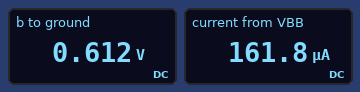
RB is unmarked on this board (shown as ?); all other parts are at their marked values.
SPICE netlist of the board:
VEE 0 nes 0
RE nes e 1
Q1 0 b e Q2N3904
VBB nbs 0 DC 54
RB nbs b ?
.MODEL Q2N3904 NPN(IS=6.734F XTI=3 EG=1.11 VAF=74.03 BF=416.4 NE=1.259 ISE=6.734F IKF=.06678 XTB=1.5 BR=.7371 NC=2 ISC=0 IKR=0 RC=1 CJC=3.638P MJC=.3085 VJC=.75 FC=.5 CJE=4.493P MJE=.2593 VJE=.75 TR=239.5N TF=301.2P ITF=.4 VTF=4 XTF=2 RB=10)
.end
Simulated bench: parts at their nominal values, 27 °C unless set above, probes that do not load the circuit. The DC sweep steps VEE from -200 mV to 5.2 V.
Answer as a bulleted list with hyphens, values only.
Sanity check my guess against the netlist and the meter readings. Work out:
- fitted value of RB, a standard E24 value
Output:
- 330 kΩ
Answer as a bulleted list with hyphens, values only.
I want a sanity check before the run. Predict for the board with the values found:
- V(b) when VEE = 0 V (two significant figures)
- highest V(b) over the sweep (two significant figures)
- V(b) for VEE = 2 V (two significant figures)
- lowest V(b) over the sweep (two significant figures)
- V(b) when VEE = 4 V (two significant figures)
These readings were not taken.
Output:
- 610 mV
- 610 mV
- -1.2 V
- -4.4 V
- -3.2 V
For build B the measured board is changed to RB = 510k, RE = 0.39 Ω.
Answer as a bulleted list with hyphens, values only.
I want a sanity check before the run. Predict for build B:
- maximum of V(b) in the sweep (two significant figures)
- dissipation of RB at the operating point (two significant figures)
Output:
- 600 mV
- 5.6 mW
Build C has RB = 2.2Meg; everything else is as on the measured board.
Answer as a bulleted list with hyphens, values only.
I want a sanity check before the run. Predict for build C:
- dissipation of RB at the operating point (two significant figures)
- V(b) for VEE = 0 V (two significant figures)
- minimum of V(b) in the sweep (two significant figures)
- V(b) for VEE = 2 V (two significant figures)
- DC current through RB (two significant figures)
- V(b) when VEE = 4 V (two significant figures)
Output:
- 1.3 mW
- 560 mV
- -4.5 V
- -1.3 V
- 24 µA
- -3.3 V
